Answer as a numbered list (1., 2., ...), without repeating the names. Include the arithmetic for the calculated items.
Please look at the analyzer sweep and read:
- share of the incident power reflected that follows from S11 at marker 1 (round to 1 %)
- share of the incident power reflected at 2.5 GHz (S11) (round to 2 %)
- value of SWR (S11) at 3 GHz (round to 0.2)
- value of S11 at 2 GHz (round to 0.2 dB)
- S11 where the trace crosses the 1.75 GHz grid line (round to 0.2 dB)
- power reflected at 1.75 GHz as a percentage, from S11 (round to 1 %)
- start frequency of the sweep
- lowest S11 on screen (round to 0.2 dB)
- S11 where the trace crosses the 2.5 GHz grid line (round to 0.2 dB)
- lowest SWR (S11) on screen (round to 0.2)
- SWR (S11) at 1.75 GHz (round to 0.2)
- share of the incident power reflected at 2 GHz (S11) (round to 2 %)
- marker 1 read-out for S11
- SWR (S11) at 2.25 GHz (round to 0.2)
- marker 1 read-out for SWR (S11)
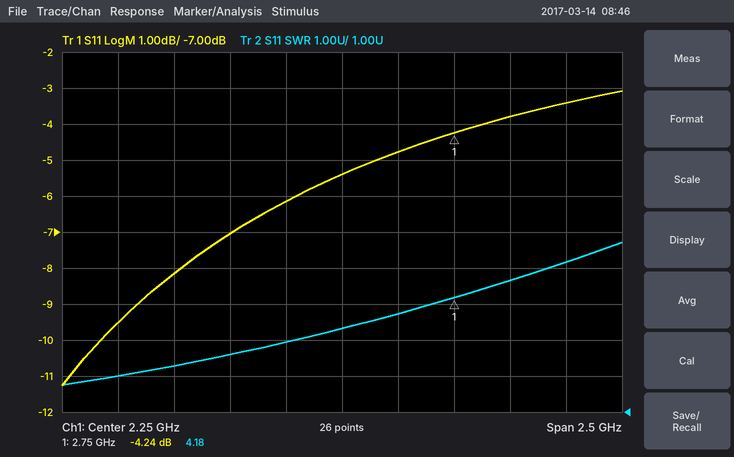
1. 10^(-4.24/10) ≈ 38 %
2. 10^(-4.8/10) ≈ 33.1 %, so 34 % to the nearest 2 %
3. 4.6
4. -6.2 dB
5. -7.0 dB
6. 10^(-7/10) ≈ 20 %
7. 1 GHz
8. -11.2 dB
9. -4.8 dB
10. 1.8
11. 2.6
12. 10^(-6.2/10) ≈ 24 %
13. -4.24 dB
14. 3.4
15. 4.18
